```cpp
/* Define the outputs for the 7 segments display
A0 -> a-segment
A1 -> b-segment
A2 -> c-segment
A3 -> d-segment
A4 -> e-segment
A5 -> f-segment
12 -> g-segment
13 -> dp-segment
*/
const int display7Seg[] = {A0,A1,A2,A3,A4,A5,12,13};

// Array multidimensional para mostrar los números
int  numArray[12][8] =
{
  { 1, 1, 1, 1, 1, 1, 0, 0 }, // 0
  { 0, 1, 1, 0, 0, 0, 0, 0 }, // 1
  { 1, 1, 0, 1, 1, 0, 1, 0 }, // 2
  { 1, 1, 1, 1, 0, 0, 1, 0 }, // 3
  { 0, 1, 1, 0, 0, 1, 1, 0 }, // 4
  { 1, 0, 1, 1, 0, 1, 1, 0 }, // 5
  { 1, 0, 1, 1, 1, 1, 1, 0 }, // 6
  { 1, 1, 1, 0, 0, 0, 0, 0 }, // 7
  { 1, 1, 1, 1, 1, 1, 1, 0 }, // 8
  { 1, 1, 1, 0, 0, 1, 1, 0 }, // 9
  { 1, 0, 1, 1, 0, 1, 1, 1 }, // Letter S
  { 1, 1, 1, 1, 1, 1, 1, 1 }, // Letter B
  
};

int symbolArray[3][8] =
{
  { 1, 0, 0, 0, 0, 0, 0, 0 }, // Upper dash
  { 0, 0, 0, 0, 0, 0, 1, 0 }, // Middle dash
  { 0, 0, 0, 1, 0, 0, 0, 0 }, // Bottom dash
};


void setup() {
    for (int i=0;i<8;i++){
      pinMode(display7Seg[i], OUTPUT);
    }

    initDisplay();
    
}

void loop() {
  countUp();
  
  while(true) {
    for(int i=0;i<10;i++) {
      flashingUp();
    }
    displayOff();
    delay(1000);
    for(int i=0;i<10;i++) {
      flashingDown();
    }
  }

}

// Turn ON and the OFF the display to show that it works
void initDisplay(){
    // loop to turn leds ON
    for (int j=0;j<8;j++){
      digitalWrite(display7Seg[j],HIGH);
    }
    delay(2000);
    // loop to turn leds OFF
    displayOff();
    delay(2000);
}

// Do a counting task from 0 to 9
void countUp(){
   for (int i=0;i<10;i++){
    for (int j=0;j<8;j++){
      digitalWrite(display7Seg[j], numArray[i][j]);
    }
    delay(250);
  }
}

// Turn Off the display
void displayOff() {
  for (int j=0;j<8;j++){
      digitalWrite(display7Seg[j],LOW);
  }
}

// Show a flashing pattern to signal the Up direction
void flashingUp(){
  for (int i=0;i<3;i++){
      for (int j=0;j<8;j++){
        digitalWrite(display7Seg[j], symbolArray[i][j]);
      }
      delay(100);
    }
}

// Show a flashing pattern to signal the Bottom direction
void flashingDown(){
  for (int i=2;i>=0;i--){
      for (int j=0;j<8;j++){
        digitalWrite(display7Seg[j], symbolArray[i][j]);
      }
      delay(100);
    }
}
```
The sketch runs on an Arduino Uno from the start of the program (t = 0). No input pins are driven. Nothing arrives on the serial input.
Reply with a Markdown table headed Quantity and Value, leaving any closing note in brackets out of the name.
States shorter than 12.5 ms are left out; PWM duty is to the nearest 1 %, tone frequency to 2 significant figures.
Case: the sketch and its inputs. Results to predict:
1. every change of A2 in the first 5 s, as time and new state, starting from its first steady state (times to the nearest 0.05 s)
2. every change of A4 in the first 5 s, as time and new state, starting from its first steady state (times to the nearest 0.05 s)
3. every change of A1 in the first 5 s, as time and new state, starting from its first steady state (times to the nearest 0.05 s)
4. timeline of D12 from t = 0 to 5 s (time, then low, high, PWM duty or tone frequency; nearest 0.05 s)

| Quantity | Value |
|---|---|
| every change of A2 in the first 5 s, as time and new state, starting from its first steady state | 0 s high; 2 s low; 4 s high; 4.5 s low; 4.75 s high |
| every change of A4 in the first 5 s, as time and new state, starting from its first steady state | 0 s high; 2 s low; 4 s high; 4.25 s low; 4.5 s high; 4.75 s low |
| every change of A1 in the first 5 s, as time and new state, starting from its first steady state | 0 s high; 2 s low; 4 s high |
| timeline of D12 from t = 0 to 5 s | 0 s high; 2 s low; 4.5 s high |
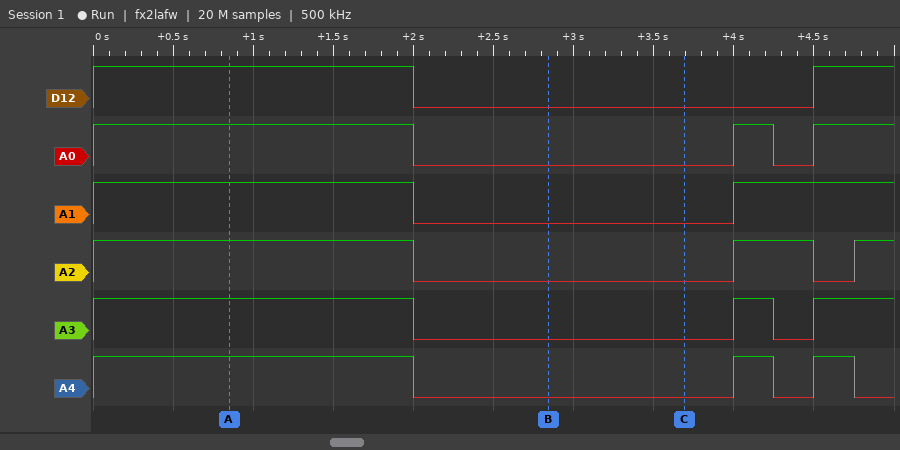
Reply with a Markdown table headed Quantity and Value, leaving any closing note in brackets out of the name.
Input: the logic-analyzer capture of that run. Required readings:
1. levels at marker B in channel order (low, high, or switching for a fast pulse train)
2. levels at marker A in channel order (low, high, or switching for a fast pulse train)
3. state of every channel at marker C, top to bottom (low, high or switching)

| Quantity | Value |
|---|---|
| levels at marker B in channel order | D12 low, A0 low, A1 low, A2 low, A3 low, A4 low |
| levels at marker A in channel order | D12 high, A0 high, A1 high, A2 high, A3 high, A4 high |
| state of every channel at marker C, top to bottom | D12 low, A0 low, A1 low, A2 low, A3 low, A4 low |
